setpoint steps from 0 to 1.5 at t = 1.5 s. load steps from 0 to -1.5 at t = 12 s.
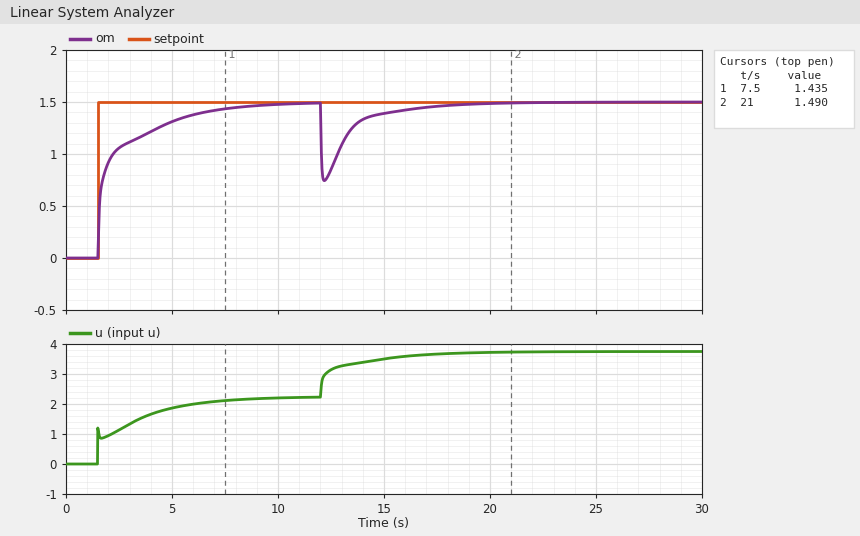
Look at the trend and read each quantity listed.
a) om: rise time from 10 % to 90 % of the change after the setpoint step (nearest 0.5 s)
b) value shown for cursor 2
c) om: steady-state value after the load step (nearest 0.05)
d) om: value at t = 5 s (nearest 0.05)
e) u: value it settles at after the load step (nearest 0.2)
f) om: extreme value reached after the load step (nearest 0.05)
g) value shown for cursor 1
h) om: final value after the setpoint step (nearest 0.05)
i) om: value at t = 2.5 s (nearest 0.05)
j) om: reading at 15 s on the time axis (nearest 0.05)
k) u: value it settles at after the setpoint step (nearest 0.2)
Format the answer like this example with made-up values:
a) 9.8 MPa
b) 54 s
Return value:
a) 4.0 s
b) 1.490
c) 1.50
d) 1.30
e) 3.8
f) 0.75
g) 1.435
h) 1.50
i) 1.05
j) 1.40
k) 2.2
